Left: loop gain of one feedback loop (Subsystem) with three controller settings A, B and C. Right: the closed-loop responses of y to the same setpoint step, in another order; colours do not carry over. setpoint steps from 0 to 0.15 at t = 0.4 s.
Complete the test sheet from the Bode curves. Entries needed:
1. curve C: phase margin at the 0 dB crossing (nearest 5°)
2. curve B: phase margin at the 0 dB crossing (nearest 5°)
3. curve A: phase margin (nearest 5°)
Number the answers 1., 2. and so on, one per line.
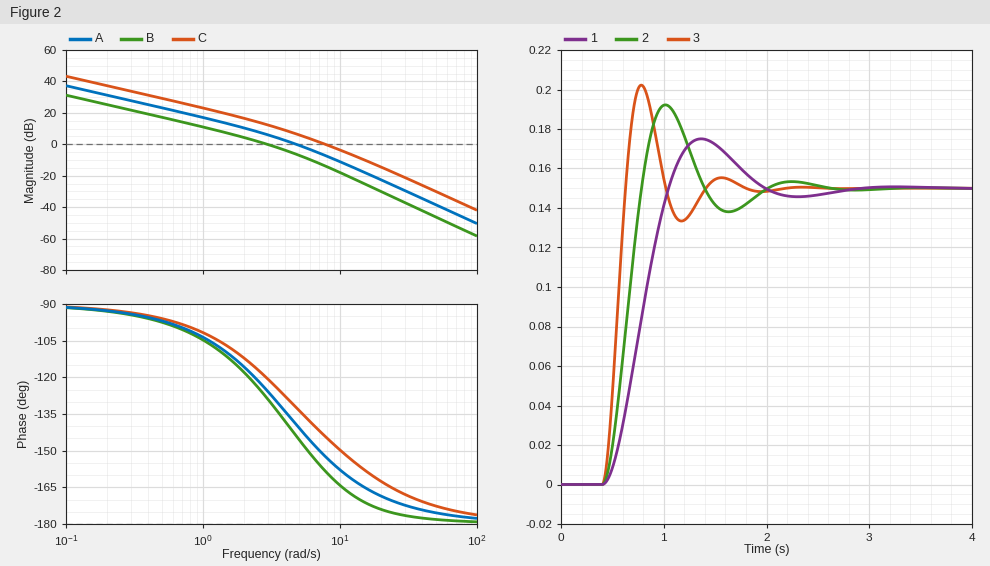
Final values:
1. 35°
2. 50°
3. 40°
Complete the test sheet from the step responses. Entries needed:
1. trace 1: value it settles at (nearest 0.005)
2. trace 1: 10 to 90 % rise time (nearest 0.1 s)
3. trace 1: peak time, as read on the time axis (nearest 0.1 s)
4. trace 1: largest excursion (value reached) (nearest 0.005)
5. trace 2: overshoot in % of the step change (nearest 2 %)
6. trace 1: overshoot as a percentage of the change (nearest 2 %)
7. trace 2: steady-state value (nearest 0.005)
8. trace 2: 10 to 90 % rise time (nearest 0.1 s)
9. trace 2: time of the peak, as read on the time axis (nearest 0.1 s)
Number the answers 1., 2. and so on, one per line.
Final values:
1. 0.150
2. 0.4 s
3. 1.4 s
4. 0.175
5. 28 %
6. 16 %
7. 0.150
8. 0.3 s
9. 1.0 s
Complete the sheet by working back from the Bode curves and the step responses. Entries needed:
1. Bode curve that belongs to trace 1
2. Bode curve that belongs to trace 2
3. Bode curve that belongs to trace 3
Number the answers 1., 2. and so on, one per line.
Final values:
1. B
2. A
3. C
